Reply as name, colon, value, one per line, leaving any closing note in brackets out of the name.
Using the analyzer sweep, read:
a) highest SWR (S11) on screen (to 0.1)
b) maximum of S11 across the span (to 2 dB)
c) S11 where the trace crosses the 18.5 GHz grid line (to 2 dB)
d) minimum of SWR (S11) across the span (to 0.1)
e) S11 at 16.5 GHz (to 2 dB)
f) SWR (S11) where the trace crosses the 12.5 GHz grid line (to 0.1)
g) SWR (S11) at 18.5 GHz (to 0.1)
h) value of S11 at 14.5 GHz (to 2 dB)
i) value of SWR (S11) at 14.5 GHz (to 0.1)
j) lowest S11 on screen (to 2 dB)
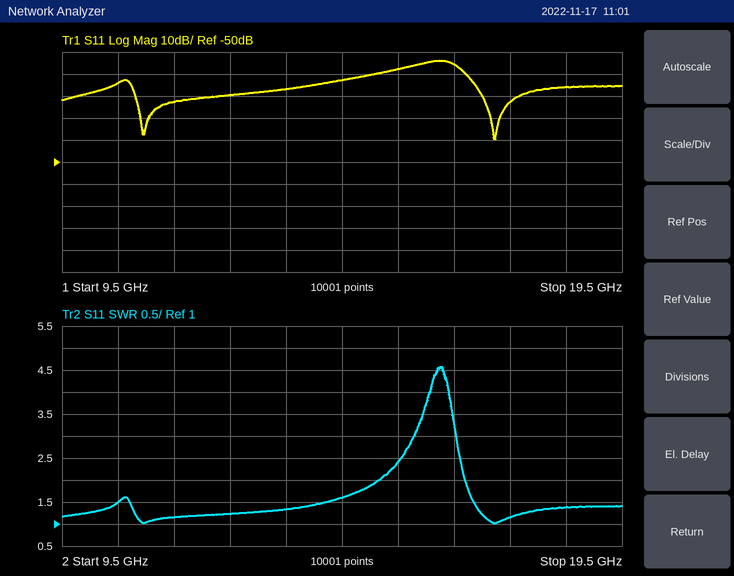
highest SWR (S11) on screen: 4.6
maximum of S11 across the span: -4 dB
S11 where the trace crosses the 18.5 GHz grid line: -16 dB
minimum of SWR (S11) across the span: 1.0
S11 at 16.5 GHz: -6 dB
SWR (S11) where the trace crosses the 12.5 GHz grid line: 1.2
SWR (S11) at 18.5 GHz: 1.4
value of S11 at 14.5 GHz: -12 dB
value of SWR (S11) at 14.5 GHz: 1.6
lowest S11 on screen: -40 dB
